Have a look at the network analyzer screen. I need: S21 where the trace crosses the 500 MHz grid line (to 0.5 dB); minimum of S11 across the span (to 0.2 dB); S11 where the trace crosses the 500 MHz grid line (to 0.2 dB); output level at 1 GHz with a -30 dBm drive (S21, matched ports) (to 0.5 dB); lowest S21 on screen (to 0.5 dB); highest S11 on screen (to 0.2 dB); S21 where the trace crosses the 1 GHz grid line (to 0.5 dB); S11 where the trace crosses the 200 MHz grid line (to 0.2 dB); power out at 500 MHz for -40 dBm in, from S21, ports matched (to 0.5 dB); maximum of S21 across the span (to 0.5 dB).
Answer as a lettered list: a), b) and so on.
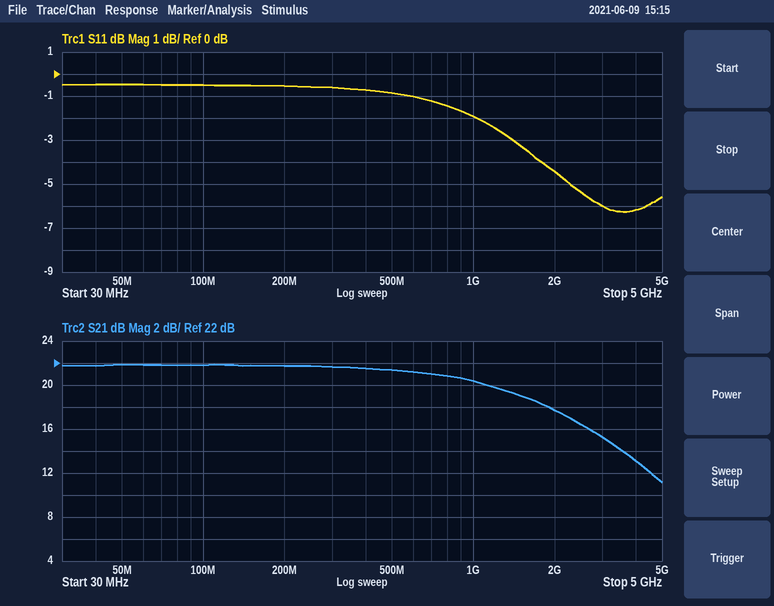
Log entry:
a) 21.5 dB
b) -6.2 dB
c) -0.8 dB
d) -9.5 dBm
e) 11.0 dB
f) -0.4 dB
g) 20.5 dB
h) -0.6 dB
i) -18.5 dBm
j) 22.0 dB
